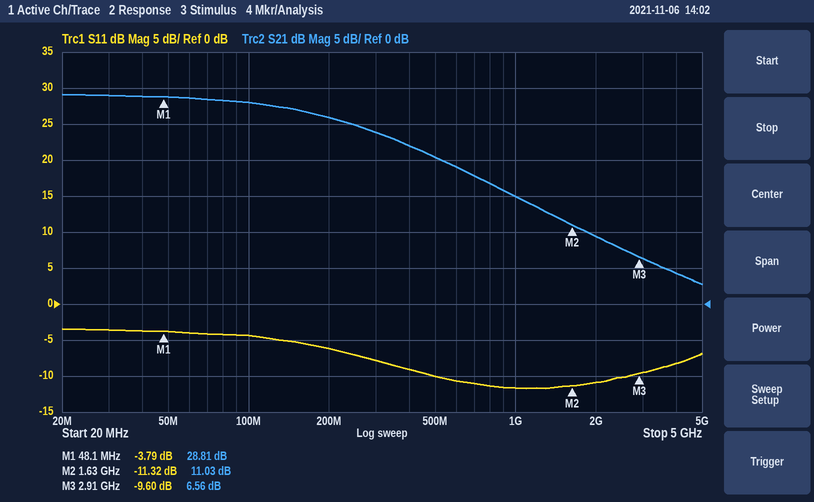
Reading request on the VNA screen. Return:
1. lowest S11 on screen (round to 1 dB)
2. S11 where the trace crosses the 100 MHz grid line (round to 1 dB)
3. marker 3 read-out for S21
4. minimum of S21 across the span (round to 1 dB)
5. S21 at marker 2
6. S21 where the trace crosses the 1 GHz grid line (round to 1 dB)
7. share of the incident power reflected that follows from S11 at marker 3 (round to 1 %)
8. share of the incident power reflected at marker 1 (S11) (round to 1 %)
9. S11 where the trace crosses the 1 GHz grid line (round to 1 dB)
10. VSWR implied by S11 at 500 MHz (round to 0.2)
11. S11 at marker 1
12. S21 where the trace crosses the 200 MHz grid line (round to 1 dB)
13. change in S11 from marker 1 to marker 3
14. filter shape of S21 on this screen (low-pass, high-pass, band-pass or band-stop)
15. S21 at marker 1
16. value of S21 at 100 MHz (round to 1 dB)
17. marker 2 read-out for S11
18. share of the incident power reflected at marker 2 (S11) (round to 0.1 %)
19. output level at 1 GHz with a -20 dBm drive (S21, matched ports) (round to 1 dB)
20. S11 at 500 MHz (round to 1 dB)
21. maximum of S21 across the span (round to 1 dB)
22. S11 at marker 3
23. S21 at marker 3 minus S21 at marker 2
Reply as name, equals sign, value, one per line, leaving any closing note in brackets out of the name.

lowest S11 on screen = -12 dB
S11 where the trace crosses the 100 MHz grid line = -4 dB
marker 3 read-out for S21 = 6.56 dB
minimum of S21 across the span = 3 dB
S21 at marker 2 = 11.03 dB
S21 where the trace crosses the 1 GHz grid line = 15 dB
share of the incident power reflected that follows from S11 at marker 3 = 11 %
share of the incident power reflected at marker 1 (S11) = 42 %
S11 where the trace crosses the 1 GHz grid line = -12 dB
VSWR implied by S11 at 500 MHz = 2.0
S11 at marker 1 = -3.79 dB
S21 where the trace crosses the 200 MHz grid line = 26 dB
change in S11 from marker 1 to marker 3 = -5.81 dB
filter shape of S21 on this screen = low-pass
S21 at marker 1 = 28.81 dB
value of S21 at 100 MHz = 28 dB
marker 2 read-out for S11 = -11.32 dB
share of the incident power reflected at marker 2 (S11) = 7.4 %
output level at 1 GHz with a -20 dBm drive (S21, matched ports) = -5 dBm
S11 at 500 MHz = -10 dB
maximum of S21 across the span = 29 dB
S11 at marker 3 = -9.60 dB
S21 at marker 3 minus S21 at marker 2 = -4.47 dB
